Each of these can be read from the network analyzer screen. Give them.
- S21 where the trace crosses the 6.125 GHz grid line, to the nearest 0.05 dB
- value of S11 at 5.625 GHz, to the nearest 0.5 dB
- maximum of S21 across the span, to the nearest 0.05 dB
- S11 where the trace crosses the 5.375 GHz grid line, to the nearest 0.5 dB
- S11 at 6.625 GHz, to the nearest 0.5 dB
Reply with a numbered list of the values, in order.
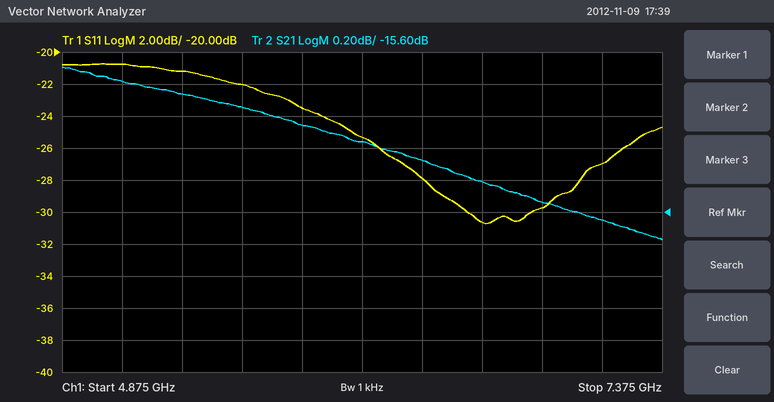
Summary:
1. -15.15 dB
2. -22.0 dB
3. -14.70 dB
4. -21.0 dB
5. -30.5 dB
